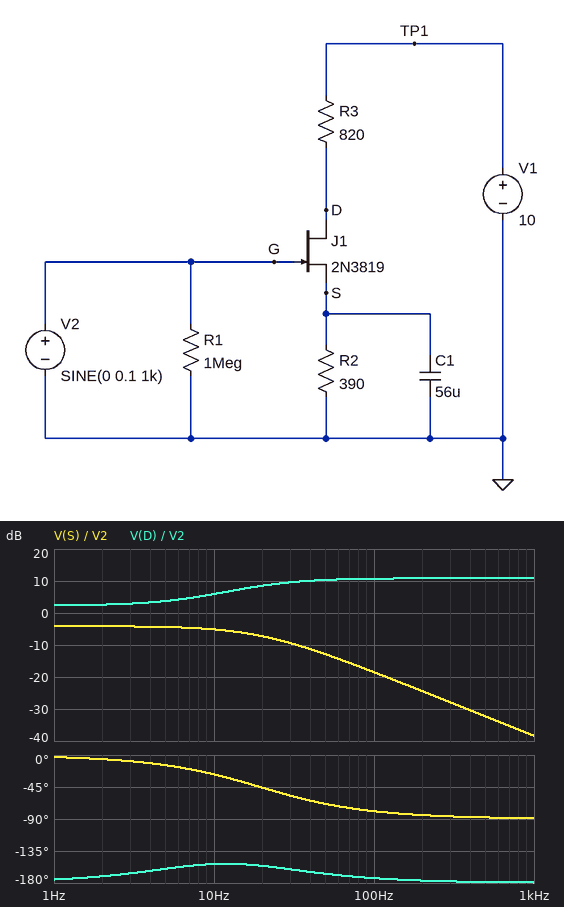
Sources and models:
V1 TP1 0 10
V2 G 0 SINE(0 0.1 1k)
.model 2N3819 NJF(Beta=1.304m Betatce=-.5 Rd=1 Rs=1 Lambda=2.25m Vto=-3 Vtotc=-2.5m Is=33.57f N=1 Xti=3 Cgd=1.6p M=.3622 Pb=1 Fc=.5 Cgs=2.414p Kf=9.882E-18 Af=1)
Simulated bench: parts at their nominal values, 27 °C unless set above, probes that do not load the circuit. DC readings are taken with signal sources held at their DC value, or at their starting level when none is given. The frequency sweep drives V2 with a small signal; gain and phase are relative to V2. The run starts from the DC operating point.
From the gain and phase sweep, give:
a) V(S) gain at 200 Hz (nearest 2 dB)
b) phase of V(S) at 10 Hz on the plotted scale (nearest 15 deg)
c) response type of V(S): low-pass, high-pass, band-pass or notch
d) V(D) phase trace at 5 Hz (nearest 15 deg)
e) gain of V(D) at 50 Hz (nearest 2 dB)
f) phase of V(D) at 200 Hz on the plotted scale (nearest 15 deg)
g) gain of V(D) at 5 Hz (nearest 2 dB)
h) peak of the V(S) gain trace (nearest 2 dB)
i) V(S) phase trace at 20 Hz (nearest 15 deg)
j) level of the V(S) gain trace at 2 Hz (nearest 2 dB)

-24 dB
-30 deg
low-pass
-165 deg
10 dB
-180 deg
4 dB
-4 dB
-45 deg
-4 dB
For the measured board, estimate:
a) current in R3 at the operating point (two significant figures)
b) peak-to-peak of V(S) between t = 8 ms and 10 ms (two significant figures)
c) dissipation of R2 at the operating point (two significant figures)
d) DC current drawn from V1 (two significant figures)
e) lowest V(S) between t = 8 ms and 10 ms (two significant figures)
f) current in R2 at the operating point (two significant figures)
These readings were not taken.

3.5 mA
2.4 mV
4.8 mW
3.5 mA
1.4 V
3.5 mA
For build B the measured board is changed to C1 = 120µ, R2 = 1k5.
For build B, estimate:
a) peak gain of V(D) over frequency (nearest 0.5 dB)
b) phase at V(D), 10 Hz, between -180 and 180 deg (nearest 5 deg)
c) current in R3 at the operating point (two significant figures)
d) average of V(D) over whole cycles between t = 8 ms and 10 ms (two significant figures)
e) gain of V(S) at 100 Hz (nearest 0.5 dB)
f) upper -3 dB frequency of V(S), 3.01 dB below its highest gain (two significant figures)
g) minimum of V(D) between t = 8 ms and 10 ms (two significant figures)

6.5 dB
-160 deg
1.3 mA
8.9 V
-29.0 dB
4.4 Hz
8.7 V
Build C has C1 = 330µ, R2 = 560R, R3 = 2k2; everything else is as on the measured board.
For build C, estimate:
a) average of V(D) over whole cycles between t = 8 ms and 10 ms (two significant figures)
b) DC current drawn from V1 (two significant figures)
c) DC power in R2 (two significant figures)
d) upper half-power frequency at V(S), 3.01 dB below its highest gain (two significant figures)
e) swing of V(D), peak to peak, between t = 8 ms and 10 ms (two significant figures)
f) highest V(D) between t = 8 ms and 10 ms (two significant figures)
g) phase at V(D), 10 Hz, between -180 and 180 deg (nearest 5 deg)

3.9 V
2.8 mA
4.3 mW
2.7 Hz
1.6 V
4.7 V
-170 deg
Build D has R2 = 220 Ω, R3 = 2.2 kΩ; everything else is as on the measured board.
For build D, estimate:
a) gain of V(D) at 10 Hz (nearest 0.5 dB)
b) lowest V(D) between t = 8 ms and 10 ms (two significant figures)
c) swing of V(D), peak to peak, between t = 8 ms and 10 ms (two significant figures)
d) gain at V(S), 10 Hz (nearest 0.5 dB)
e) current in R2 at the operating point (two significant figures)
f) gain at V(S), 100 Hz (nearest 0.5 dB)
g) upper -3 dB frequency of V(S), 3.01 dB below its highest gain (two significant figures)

-6.0 dB
1.6 V
110 mV
-28.0 dB
3.8 mA
-43.0 dB
15 Hz
